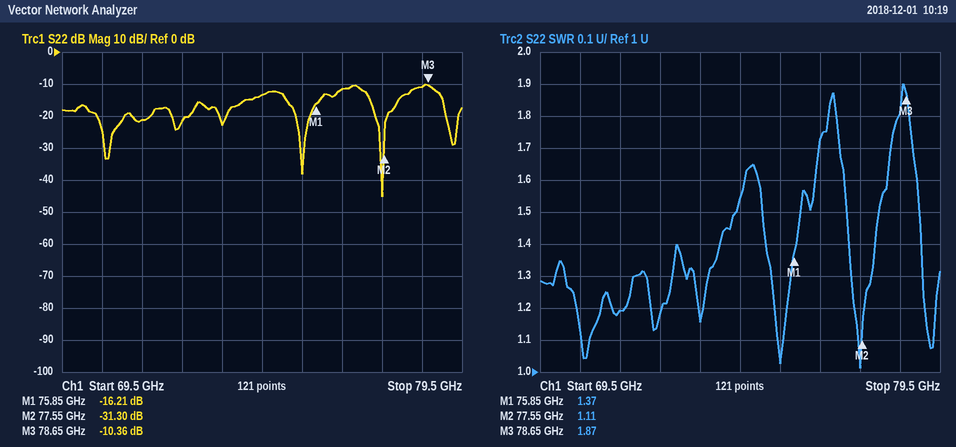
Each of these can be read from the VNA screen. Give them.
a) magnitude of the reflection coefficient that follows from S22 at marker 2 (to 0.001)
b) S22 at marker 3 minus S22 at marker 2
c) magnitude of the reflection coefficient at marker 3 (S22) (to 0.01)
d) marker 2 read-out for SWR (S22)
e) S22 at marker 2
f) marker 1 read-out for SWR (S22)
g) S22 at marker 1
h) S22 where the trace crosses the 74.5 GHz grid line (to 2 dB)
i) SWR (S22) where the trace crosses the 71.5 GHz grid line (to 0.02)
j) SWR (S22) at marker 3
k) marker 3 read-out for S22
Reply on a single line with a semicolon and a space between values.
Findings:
0.027; 20.94 dB; 0.30; 1.11; -31.30 dB; 1.37; -16.21 dB; -14 dB; 1.20; 1.87; -10.36 dB
